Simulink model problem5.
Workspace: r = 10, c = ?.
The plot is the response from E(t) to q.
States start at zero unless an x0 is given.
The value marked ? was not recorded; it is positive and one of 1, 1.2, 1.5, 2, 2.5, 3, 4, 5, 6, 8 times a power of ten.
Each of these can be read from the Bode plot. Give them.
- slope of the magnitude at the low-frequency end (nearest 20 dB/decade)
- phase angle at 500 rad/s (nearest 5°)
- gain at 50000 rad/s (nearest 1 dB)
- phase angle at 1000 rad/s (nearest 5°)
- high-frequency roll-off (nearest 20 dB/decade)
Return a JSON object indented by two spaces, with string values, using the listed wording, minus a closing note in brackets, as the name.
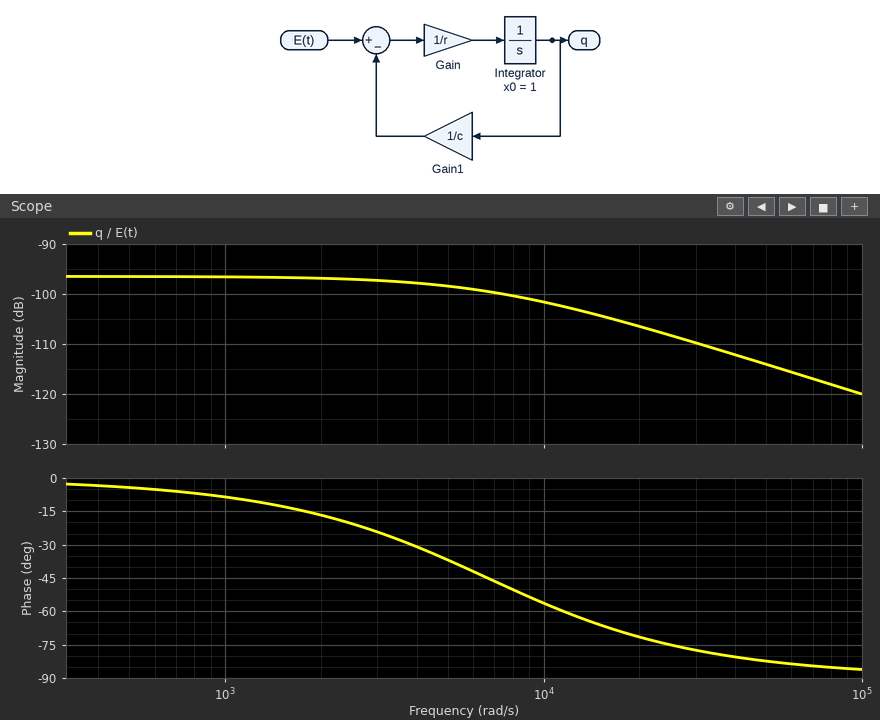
{
  "slope of the magnitude at the low-frequency end": "0 dB/decade",
  "phase angle at 500 rad/s": "-5°",
  "gain at 50000 rad/s": "-114 dB",
  "phase angle at 1000 rad/s": "-10°",
  "high-frequency roll-off": "-20 dB/decade"
}
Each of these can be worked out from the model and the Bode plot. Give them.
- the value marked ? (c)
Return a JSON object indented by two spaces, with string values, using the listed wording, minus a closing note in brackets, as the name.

{
  "the value marked ?": "1.5e-05"
}
